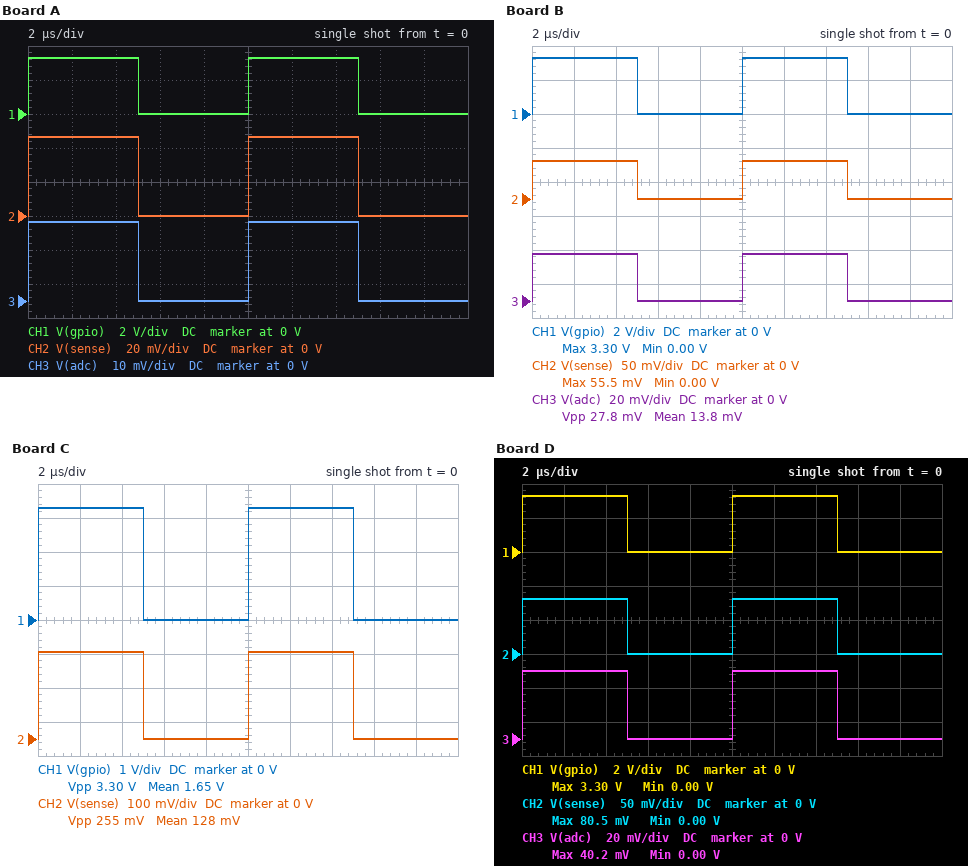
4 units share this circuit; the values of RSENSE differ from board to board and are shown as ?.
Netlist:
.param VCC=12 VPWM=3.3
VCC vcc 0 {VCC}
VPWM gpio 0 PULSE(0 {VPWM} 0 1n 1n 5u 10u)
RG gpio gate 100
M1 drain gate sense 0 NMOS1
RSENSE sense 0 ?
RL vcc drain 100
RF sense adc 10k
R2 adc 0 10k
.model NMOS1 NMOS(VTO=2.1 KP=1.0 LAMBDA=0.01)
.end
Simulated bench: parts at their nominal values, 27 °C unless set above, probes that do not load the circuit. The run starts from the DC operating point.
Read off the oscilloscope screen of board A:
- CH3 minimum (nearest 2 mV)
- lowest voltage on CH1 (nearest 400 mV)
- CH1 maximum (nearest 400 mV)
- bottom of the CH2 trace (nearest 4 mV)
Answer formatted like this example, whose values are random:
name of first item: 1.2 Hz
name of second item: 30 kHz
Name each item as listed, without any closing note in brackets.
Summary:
CH3 minimum: 0 V
lowest voltage on CH1: 0 V
CH1 maximum: 3.2 V
bottom of the CH2 trace: 0 V
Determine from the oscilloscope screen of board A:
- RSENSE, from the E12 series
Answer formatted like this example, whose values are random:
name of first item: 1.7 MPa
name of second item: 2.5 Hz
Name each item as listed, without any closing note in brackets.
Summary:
RSENSE, from the E12 series: 0.39 Ω
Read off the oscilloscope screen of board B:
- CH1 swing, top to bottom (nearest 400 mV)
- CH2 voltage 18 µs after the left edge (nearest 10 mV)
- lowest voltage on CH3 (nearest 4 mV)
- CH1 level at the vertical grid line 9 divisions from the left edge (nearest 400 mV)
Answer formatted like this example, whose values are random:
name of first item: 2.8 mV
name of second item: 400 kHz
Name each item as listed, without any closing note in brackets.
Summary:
CH1 swing, top to bottom: 3.2 V
CH2 voltage 18 µs after the left edge: 0 V
lowest voltage on CH3: 0 V
CH1 level at the vertical grid line 9 divisions from the left edge: 0 V
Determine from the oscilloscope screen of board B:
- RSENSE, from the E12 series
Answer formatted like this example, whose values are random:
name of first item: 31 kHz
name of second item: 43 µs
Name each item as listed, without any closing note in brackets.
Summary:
RSENSE, from the E12 series: 0.47 Ω
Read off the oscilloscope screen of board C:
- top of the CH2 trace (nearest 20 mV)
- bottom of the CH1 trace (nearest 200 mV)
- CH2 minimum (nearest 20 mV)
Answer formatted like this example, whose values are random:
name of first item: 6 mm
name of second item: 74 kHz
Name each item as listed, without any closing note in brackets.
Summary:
top of the CH2 trace: 260 mV
bottom of the CH1 trace: 0 V
CH2 minimum: 0 V
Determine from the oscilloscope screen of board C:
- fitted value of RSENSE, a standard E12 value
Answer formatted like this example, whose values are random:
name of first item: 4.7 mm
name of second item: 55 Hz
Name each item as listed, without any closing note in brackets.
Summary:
fitted value of RSENSE, a standard E12 value: 2.2 Ω
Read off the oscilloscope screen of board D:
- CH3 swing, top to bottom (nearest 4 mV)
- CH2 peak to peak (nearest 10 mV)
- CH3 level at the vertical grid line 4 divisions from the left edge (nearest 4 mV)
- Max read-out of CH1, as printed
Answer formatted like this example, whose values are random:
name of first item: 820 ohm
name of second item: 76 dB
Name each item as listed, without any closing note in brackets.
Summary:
CH3 swing, top to bottom: 40 mV
CH2 peak to peak: 80 mV
CH3 level at the vertical grid line 4 divisions from the left edge: 0 V
Max read-out of CH1, as printed: 3.30 V
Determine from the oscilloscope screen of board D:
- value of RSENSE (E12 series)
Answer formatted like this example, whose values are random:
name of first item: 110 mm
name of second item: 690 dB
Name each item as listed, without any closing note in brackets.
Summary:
value of RSENSE: 0.68 Ω
